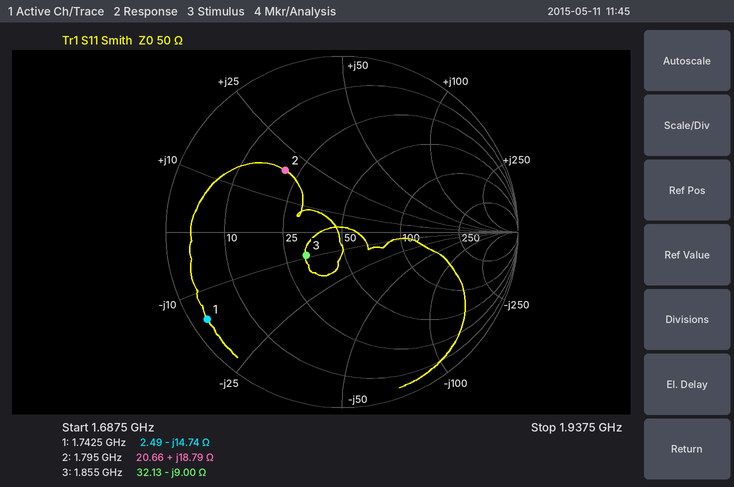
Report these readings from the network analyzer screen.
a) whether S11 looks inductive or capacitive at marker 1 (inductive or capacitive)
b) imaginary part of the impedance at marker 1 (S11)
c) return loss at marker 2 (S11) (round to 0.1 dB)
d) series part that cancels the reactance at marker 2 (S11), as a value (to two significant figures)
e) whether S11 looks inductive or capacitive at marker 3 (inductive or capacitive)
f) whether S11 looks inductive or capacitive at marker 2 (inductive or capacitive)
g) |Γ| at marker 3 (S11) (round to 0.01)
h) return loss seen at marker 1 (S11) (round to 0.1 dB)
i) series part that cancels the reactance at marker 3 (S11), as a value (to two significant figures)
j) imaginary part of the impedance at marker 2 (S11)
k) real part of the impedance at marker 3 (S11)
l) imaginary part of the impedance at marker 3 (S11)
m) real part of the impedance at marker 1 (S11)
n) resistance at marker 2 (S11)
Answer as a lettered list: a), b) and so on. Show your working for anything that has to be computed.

a) capacitive
b) -14.74 Ω
c) 6.4 dB
d) C = 1/(2π × 1.795 GHz × 18.79 Ω) ≈ 4.7 pF
e) capacitive
f) inductive
g) 0.24
h) 0.8 dB
i) L = 9 Ω/(2π × 1.855 GHz) ≈ 772 pH, so 770 pH to two significant figures
j) +18.79 Ω
k) 32.13 Ω
l) -9.00 Ω
m) 2.49 Ω
n) 20.66 Ω
